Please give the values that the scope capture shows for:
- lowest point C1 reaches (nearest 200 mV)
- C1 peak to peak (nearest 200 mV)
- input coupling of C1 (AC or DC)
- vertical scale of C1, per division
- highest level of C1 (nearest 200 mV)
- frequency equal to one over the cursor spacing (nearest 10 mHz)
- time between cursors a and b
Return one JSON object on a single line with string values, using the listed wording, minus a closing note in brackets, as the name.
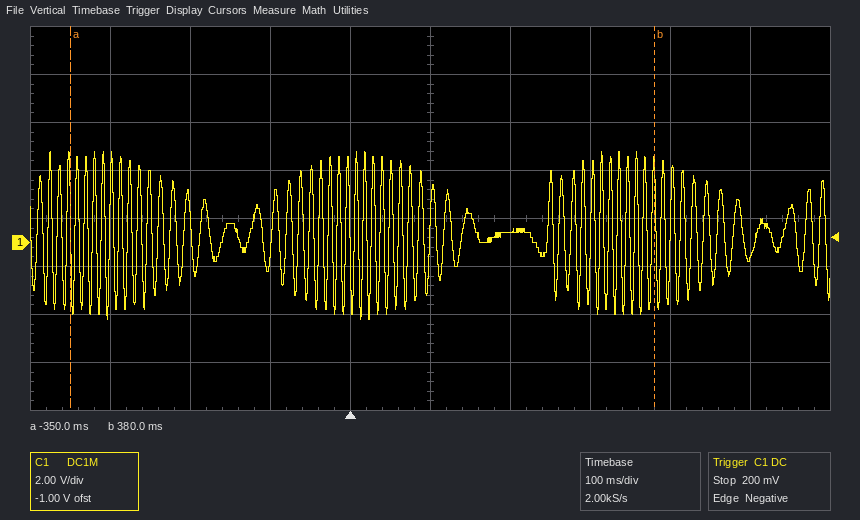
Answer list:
{"lowest point C1 reaches": "-3.2 V", "C1 peak to peak": "7.0 V", "input coupling of C1": "DC", "vertical scale of C1, per division": "2 V", "highest level of C1": "3.8 V", "frequency equal to one over the cursor spacing": "1.37 Hz", "time between cursors a and b": "730 ms"}
